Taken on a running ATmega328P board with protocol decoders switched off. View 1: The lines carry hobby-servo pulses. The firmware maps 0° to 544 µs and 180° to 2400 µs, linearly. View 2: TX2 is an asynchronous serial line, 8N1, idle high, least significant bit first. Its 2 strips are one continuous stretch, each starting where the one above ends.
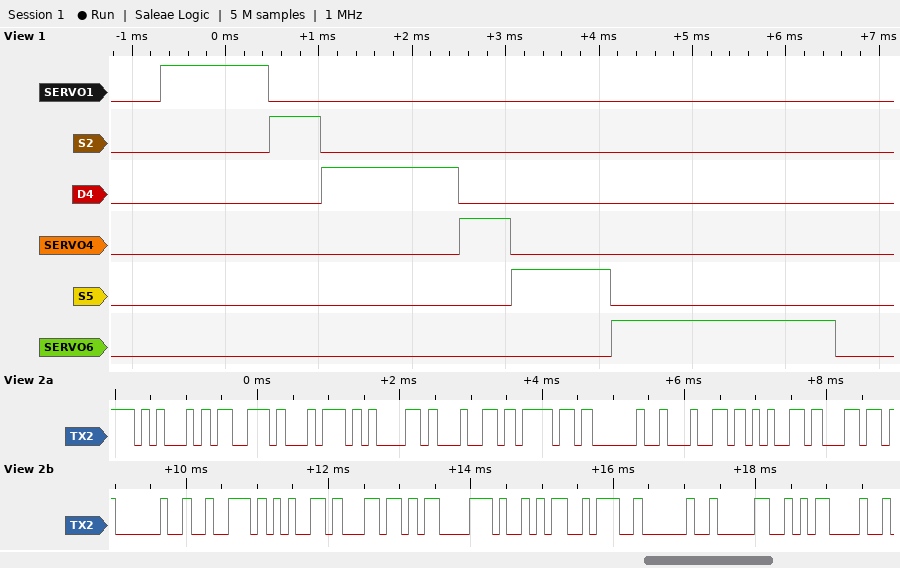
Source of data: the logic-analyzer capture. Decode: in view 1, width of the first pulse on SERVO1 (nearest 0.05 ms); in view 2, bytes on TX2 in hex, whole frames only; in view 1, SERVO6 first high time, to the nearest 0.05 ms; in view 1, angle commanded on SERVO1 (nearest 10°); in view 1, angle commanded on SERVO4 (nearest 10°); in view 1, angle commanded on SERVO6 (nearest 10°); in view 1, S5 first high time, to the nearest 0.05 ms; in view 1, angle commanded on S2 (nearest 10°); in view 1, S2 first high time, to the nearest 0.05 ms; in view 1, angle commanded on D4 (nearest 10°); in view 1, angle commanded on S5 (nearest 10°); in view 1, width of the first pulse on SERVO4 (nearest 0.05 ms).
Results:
1.15 ms
45 73 74 61 64 6F 20 64 65 6C 20 72 65 6C C3 A9 3A 20 30 0D
2.40 ms
60°
0°
180°
1.05 ms
0°
0.55 ms
90°
50°
0.55 ms
